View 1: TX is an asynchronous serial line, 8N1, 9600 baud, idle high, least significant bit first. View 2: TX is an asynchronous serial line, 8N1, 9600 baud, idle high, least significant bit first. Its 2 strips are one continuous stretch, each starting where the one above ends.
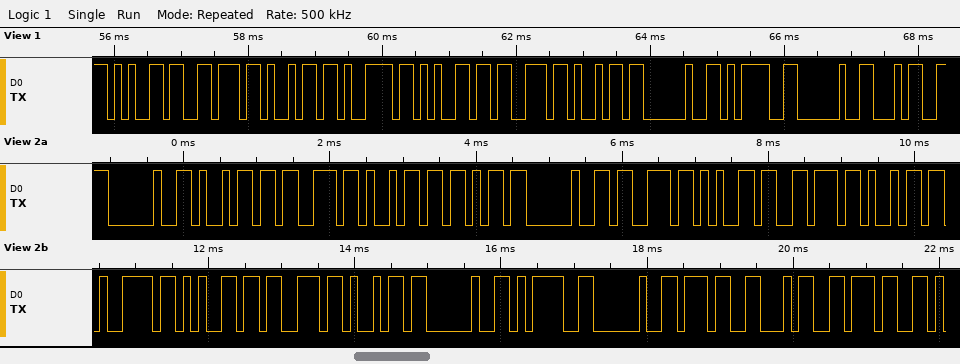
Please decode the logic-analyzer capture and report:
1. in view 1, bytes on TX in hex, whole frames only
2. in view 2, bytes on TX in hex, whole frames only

65 76 69 79 65 73 69 20 3D 20 34
0x20 0x69 0x73 0x69 0x6B 0x20 0x73 0x65 0x76 0x69 0x79 0x65 0x73 0x69 0x20 0x3D 0x20 0x37 0x34 0x37
